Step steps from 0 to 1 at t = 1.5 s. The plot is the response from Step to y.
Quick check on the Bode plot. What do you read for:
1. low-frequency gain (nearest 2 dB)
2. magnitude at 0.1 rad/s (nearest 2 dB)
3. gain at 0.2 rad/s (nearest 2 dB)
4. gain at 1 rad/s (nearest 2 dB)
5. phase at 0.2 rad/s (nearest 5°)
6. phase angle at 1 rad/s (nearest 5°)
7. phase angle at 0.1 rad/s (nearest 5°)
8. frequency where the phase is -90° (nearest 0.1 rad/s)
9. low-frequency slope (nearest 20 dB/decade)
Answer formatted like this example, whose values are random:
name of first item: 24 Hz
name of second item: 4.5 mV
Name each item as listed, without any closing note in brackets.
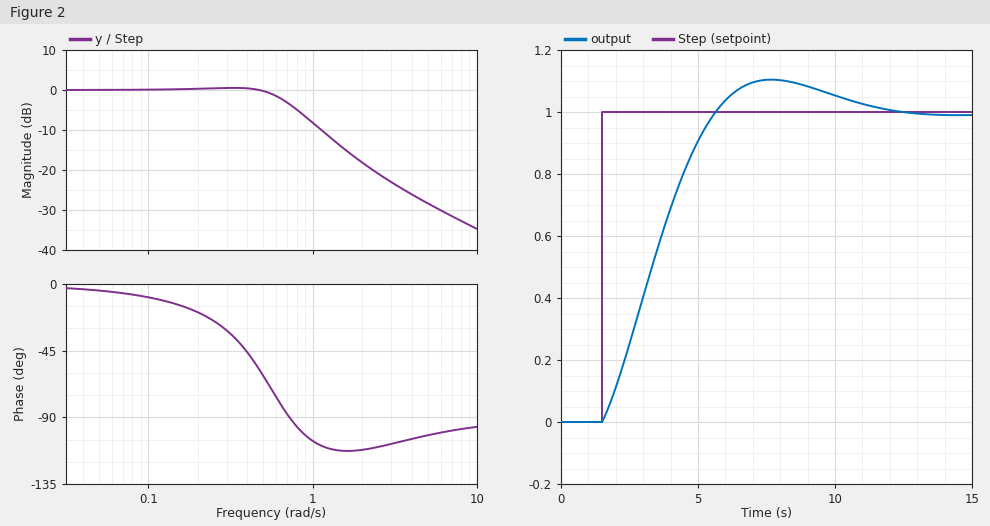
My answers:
low-frequency gain: 0 dB
magnitude at 0.1 rad/s: 0 dB
gain at 0.2 rad/s: 0 dB
gain at 1 rad/s: -8 dB
phase at 0.2 rad/s: -20°
phase angle at 1 rad/s: -105°
phase angle at 0.1 rad/s: -10°
frequency where the phase is -90°: 0.7 rad/s
low-frequency slope: 0 dB/decade
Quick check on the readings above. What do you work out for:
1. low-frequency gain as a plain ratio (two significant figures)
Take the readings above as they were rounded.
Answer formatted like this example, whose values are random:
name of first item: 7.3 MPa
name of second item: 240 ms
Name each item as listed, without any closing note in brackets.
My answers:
low-frequency gain as a plain ratio: 1.0
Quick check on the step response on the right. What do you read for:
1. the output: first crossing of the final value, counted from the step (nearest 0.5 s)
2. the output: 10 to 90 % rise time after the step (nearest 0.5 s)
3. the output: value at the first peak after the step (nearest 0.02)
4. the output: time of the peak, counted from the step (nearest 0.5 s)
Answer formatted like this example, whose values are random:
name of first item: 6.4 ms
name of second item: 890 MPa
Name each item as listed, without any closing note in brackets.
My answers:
the output: first crossing of the final value, counted from the step: 4.0 s
the output: 10 to 90 % rise time after the step: 3.0 s
the output: value at the first peak after the step: 1.10
the output: time of the peak, counted from the step: 6.0 s
